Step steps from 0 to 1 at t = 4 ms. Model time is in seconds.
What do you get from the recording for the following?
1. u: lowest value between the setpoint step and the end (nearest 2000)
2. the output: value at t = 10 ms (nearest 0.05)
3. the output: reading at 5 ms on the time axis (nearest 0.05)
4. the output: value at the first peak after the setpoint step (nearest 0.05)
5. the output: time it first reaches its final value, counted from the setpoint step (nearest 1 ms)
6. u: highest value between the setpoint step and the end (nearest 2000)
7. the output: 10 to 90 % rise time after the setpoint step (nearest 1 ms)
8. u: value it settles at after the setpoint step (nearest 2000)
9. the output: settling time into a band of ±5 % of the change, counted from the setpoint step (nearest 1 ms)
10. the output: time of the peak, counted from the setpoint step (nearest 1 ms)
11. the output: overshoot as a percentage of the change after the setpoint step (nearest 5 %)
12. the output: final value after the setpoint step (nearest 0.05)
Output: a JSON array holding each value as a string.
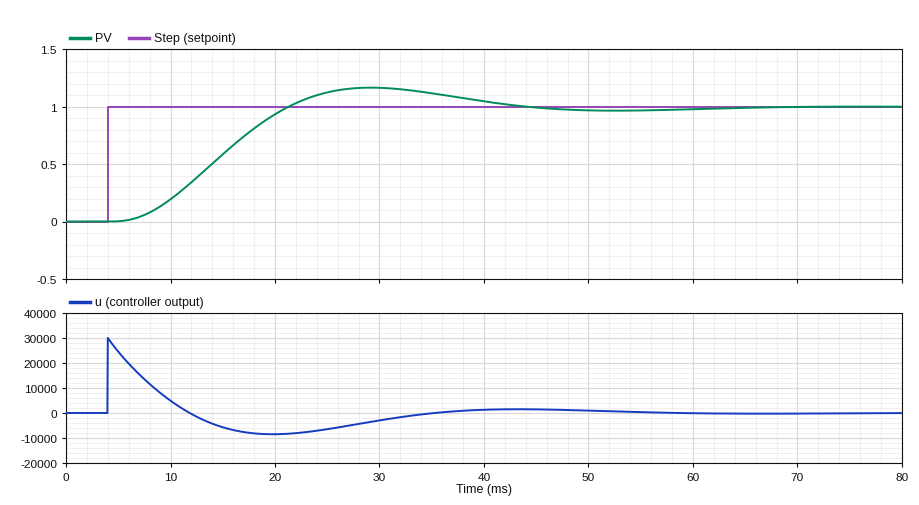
["-8000", "0.20", "0.00", "1.15", "17 ms", "30000", "11 ms", "0", "36 ms", "25 ms", "15 %", "1.00"]
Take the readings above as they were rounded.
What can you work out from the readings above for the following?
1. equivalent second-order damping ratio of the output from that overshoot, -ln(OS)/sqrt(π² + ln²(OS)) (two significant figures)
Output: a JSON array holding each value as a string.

["0.52"]
